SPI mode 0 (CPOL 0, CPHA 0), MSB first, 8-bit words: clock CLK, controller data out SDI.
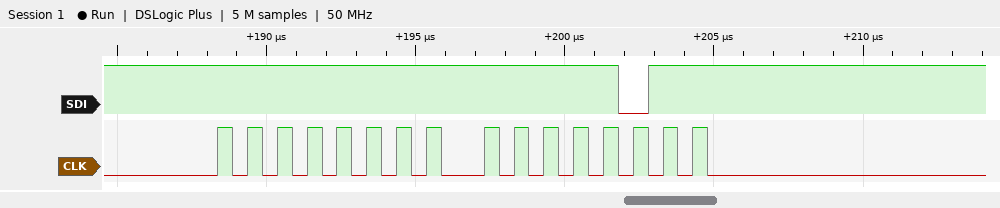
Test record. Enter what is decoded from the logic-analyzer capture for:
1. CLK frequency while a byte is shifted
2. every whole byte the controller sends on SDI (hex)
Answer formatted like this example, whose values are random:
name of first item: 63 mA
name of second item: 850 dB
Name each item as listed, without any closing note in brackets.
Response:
CLK frequency while a byte is shifted: 1 MHz
every whole byte the controller sends on SDI: 0xFF 0xFB
